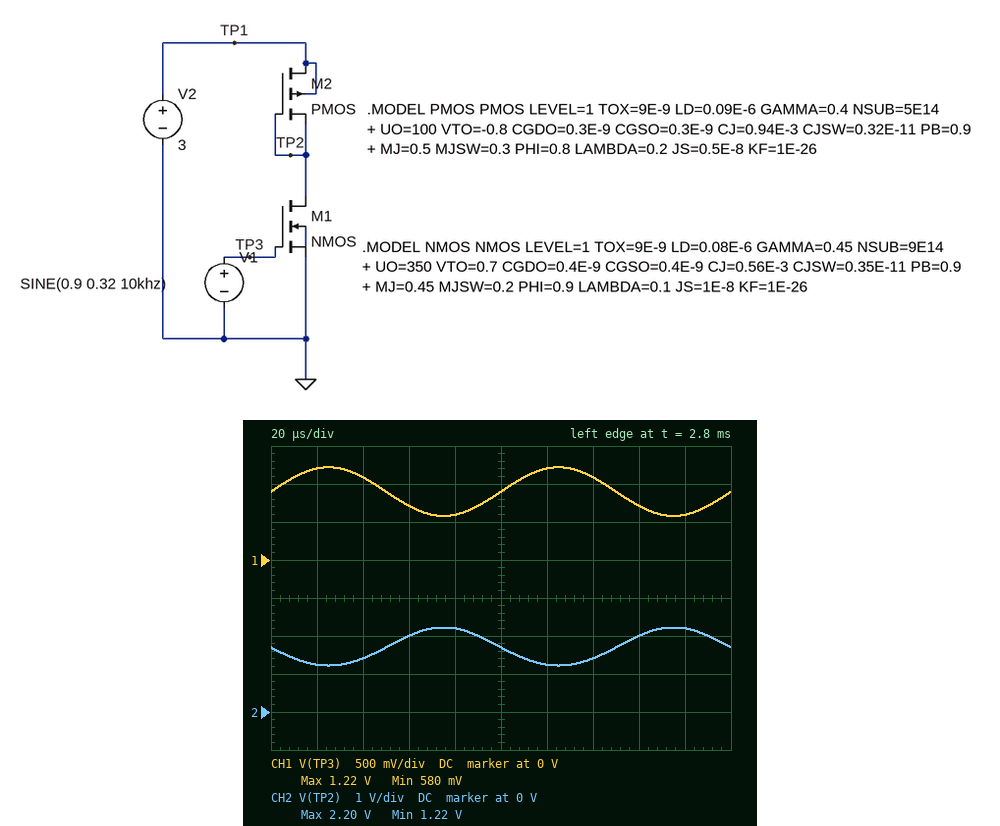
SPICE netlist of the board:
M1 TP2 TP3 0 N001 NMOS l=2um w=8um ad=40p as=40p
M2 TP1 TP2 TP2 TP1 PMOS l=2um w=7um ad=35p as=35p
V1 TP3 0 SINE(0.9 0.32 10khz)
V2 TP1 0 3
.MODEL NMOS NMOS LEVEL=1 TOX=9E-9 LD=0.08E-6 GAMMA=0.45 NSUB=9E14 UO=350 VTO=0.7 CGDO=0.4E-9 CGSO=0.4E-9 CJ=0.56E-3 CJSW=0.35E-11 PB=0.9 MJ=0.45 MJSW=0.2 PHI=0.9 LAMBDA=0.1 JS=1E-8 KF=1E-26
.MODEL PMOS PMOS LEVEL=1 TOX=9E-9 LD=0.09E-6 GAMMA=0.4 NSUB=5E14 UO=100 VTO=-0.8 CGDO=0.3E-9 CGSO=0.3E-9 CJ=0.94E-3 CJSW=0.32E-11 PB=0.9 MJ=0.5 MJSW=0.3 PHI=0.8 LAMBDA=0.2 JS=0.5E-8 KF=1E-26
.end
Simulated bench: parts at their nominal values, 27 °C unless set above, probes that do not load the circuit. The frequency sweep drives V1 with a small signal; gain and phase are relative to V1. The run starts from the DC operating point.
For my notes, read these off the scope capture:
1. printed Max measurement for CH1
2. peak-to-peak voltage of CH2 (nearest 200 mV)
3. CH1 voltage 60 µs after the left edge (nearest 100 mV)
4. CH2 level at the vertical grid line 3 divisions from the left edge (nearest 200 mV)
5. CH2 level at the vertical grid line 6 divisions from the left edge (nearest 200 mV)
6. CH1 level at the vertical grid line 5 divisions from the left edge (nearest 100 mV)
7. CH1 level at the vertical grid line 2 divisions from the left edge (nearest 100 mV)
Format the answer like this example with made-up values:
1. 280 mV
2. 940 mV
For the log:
1. 1.22 V
2. 1.0 V
3. 700 mV
4. 2.0 V
5. 1.2 V
6. 900 mV
7. 1.1 V
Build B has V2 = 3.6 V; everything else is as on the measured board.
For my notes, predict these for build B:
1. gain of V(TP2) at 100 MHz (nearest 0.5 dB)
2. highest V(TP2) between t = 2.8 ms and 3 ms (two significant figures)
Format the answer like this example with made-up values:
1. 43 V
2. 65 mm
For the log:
1. 3.5 dB
2. 2.8 V
